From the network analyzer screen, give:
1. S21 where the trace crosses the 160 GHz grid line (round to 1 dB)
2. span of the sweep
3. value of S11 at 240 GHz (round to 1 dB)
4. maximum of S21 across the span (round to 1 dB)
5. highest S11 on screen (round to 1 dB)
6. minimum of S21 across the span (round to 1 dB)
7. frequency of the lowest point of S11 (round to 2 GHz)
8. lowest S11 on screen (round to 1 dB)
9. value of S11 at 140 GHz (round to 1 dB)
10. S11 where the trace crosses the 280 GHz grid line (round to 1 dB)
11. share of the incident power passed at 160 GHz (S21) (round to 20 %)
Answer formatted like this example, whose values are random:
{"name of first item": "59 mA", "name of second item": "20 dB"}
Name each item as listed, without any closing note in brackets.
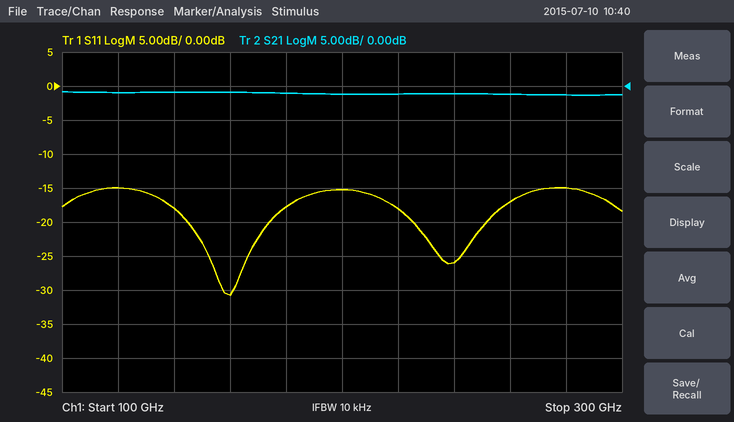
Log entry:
{"S21 where the trace crosses the 160 GHz grid line": "-1 dB", "span of the sweep": "200 GHz", "value of S11 at 240 GHz": "-26 dB", "maximum of S21 across the span": "-1 dB", "highest S11 on screen": "-15 dB", "minimum of S21 across the span": "-1 dB", "frequency of the lowest point of S11": "160 GHz", "lowest S11 on screen": "-31 dB", "value of S11 at 140 GHz": "-18 dB", "S11 where the trace crosses the 280 GHz grid line": "-15 dB", "share of the incident power passed at 160 GHz (S21)": "80 %"}
